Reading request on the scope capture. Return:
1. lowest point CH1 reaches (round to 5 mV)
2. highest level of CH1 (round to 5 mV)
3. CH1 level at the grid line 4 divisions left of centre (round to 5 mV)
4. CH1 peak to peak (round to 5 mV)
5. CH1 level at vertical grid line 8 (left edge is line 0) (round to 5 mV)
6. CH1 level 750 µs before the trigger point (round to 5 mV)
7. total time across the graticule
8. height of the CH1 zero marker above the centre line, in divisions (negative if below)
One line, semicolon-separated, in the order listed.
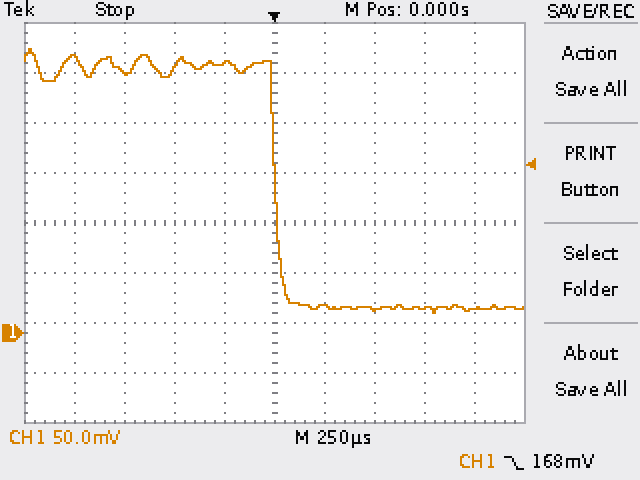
20 mV; 285 mV; 275 mV; 265 mV; 25 mV; 260 mV; 2.5 ms; -2.2 div
